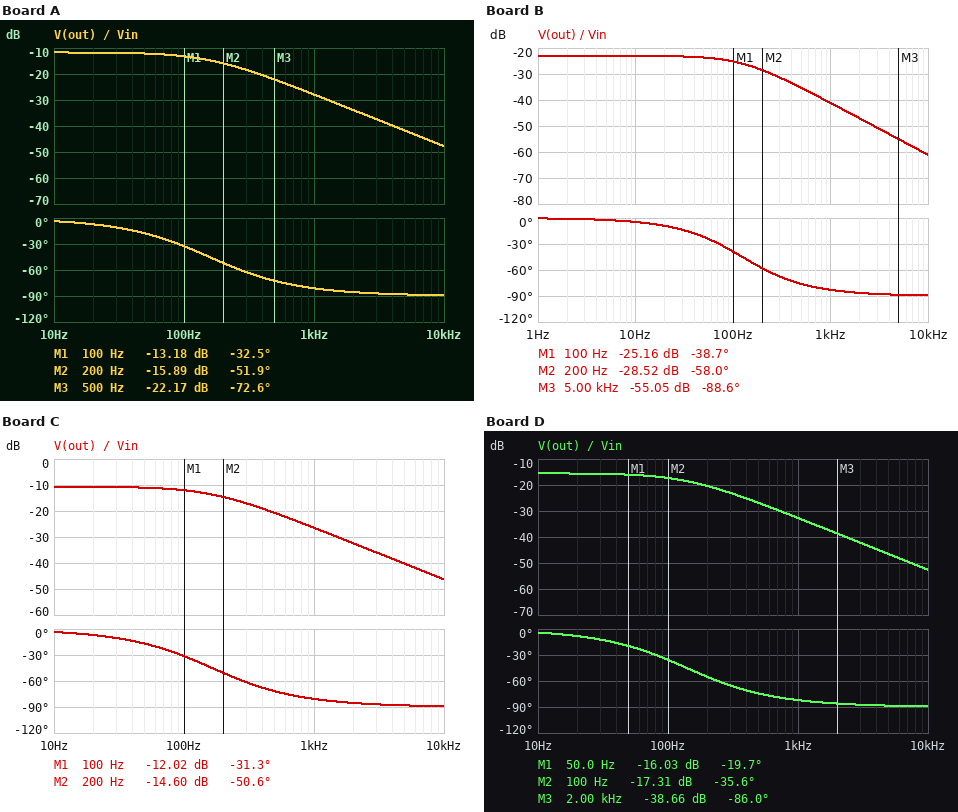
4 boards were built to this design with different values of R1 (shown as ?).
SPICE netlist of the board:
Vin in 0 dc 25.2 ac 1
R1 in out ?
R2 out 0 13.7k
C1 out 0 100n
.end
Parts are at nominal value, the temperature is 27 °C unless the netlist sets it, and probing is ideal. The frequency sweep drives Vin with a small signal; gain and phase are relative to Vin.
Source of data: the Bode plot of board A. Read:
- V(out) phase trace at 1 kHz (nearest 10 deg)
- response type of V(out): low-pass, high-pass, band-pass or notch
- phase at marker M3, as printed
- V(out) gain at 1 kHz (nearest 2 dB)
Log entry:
-80 deg
low-pass
-72.6 deg
-28 dB
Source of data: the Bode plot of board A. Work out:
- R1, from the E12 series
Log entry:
39 kΩ
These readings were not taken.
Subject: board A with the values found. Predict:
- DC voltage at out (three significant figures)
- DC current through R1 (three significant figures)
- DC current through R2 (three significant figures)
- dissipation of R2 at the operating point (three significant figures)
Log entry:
6.55 V
478 µA
478 µA
3.13 mW
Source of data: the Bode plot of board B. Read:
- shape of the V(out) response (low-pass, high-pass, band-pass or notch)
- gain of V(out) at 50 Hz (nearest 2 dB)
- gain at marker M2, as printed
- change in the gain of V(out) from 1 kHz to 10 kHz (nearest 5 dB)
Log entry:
low-pass
-24 dB
-28.52 dB
-20 dB
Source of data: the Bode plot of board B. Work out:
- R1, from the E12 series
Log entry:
180 kΩ
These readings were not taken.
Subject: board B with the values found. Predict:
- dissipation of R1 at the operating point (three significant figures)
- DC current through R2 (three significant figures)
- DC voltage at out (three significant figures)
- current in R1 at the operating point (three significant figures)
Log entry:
3.05 mW
130 µA
1.78 V
130 µA
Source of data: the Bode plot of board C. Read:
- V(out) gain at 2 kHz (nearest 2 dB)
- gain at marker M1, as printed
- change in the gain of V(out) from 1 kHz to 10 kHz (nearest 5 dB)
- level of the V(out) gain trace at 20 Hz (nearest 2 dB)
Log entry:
-32 dB
-12.02 dB
-20 dB
-10 dB
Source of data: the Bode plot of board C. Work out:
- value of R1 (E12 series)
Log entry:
33 kΩ
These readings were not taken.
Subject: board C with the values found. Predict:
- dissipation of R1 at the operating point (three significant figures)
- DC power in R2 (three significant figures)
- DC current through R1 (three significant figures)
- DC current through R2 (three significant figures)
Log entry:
9.61 mW
3.99 mW
540 µA
540 µA
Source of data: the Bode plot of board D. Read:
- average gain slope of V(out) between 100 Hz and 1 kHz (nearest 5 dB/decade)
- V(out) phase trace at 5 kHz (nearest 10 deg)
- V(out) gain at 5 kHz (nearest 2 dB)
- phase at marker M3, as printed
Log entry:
-15 dB/decade
-90 deg
-46 dB
-86.0 deg
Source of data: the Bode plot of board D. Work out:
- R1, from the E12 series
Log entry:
68 kΩ
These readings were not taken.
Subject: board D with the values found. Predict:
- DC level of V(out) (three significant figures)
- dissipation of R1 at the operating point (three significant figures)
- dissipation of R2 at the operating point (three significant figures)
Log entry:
4.23 V
6.47 mW
1.30 mW
